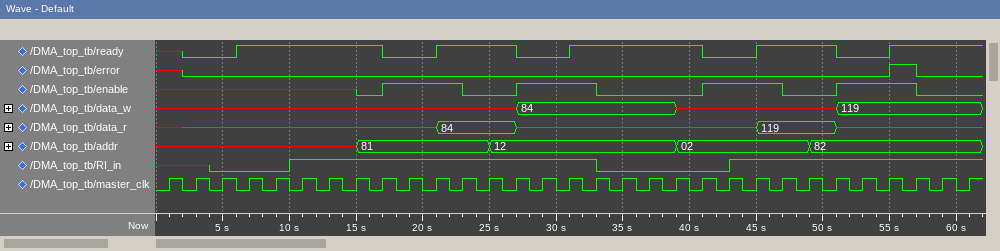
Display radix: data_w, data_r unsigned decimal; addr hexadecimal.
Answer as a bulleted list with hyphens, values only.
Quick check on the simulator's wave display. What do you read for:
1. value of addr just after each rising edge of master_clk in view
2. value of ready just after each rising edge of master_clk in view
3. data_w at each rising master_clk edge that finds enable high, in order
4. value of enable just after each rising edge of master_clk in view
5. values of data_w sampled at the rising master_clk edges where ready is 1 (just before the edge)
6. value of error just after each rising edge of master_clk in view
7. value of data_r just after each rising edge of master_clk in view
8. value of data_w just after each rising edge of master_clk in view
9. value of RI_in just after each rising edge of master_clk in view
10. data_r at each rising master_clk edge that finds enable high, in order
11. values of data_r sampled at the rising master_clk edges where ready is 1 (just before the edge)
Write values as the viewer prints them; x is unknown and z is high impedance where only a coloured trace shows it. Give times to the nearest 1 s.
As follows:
- x, x, x, x, x, x, x, 81, 81, 81, 81, 81, 12, 12, 12, 12, 12, 12, 12, 02, 02, 02, 02, 02, 82, 82, 82, 82, 82, 82, 82
- x 0 0 1 1 1 1 1 0 0 1 1 1 0 0 1 1 1 1 1 0 0 1 1 1 0 0 1 1 1 1
- x, x, x, 84, 84, 84, x, x, x, 119, 119, 119
- x x x x x x x 0 1 1 1 0 0 1 1 1 0 0 0 0 1 1 1 0 0 1 1 1 0 0 0
- x, x, x, x, x, x, x, x, x, 84, 84, 84, 84, x, x, x, x, 119, 119, 119
- x 0 0 0 0 0 0 0 0 0 0 0 0 0 0 0 0 0 0 0 0 0 0 0 0 0 0 1 0 0 0
- x, z, z, z, z, z, z, z, z, z, 84, 84, 84, z, z, z, z, z, z, z, z, z, 119, 119, 119, z, z, z, z, z, z
- x, x, x, x, x, x, x, x, x, x, x, x, x, 84, 84, 84, 84, 84, 84, x, x, x, x, x, x, 119, 119, 119, 119, 119, 119
- x x 0 0 0 1 1 1 1 1 1 1 1 1 1 1 0 0 0 0 0 1 1 1 1 1 1 1 1 1 1
- z, z, 84, z, z, z, z, z, 119, z, z, z
- z, z, z, z, z, z, 84, 84, 84, z, z, z, z, z, 119, 119, 119, z, z, z
